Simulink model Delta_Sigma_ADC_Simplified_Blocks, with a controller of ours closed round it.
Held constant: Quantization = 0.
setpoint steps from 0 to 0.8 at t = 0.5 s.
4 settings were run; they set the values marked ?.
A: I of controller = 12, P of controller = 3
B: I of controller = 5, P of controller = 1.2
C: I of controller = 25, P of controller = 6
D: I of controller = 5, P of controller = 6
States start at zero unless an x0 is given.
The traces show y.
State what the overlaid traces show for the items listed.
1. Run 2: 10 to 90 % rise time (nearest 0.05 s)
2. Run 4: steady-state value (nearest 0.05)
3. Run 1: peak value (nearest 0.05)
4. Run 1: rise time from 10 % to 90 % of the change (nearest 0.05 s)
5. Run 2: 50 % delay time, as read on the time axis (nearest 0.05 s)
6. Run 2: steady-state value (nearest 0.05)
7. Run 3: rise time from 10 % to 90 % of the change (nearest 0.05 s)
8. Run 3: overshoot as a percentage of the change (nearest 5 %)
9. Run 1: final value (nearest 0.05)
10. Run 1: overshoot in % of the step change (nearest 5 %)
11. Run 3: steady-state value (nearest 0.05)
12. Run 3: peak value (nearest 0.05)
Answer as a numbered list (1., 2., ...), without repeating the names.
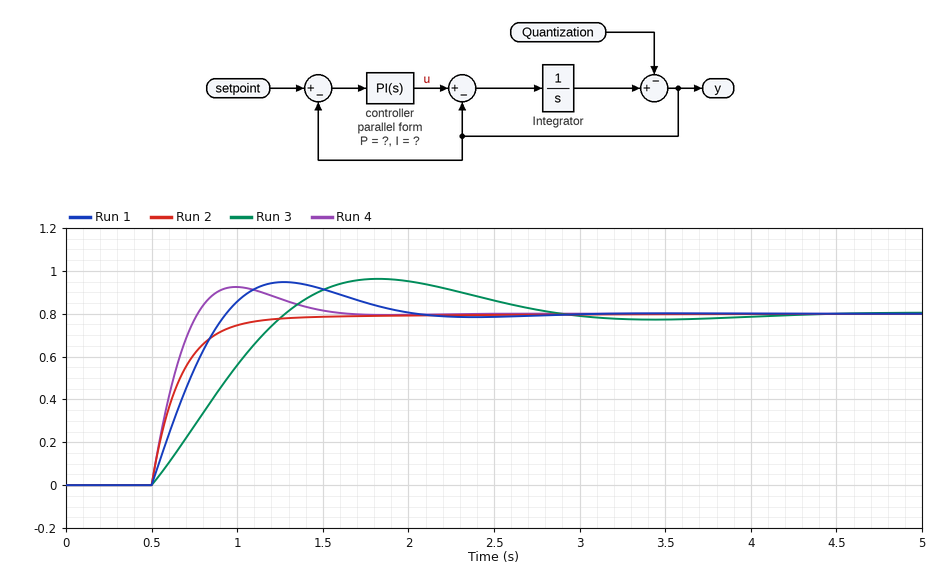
1. 0.40 s
2. 0.80
3. 0.95
4. 0.35 s
5. 0.60 s
6. 0.80
7. 0.60 s
8. 20 %
9. 0.80
10. 20 %
11. 0.80
12. 0.95
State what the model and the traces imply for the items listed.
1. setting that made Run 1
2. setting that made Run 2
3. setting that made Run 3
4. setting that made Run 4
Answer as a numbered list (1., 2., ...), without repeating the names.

1. A
2. D
3. B
4. C
